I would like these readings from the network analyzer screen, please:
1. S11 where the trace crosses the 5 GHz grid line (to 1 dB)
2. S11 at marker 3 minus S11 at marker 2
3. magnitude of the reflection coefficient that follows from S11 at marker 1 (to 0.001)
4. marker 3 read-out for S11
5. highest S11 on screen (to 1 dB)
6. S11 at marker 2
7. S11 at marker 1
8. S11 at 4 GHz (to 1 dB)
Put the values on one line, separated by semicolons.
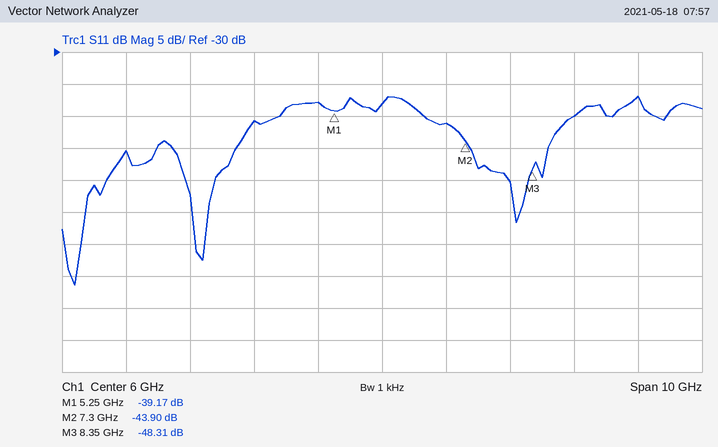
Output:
-38 dB; -4.41 dB; 0.011; -48.31 dB; -37 dB; -43.90 dB; -39.17 dB; -41 dB
